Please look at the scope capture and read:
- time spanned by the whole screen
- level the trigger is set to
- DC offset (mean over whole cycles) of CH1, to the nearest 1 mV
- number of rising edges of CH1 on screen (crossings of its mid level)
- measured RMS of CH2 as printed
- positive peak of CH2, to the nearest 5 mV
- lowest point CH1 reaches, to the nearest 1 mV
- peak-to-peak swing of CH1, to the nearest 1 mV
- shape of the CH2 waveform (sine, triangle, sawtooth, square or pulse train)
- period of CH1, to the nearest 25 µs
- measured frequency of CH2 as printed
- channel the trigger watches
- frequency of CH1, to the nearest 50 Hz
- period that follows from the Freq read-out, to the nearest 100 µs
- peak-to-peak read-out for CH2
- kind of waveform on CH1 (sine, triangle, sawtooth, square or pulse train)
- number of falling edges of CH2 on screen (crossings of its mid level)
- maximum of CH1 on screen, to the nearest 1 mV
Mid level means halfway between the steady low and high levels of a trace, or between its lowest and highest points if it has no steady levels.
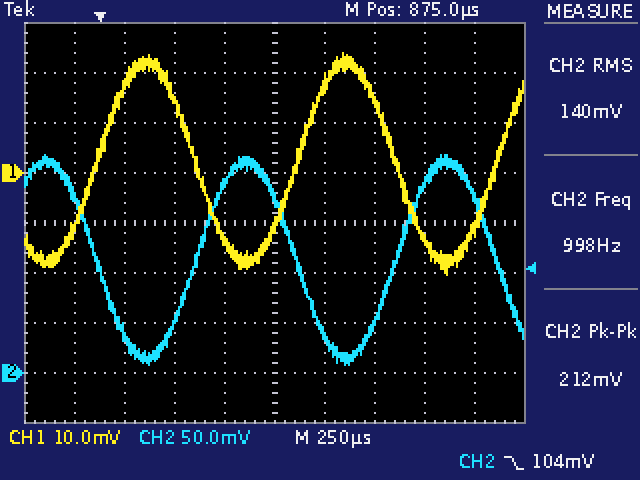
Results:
2.5 ms
104 mV
2 mV
3
140 mV
220 mV
-20 mV
44 mV
sine
1.000 ms
998 Hz
CH2
1.00 kHz
1.0 ms
212 mV
sine
3
24 mV
